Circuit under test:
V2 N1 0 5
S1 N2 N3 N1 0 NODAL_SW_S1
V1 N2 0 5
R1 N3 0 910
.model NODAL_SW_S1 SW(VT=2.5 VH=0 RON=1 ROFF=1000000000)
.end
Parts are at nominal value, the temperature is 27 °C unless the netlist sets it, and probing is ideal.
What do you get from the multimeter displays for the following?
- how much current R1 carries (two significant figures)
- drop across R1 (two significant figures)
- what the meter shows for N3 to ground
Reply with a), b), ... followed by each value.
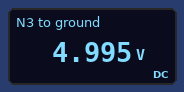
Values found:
a) 5.5 mA
b) 5.0 V
c) 4.995 V
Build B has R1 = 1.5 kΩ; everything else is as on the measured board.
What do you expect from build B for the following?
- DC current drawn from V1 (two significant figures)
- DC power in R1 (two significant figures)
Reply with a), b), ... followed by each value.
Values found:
a) 3.3 mA
b) 17 mW
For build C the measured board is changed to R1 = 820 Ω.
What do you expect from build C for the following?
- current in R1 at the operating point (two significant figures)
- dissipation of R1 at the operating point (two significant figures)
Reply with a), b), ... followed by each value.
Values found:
a) 6.1 mA
b) 30 mW
